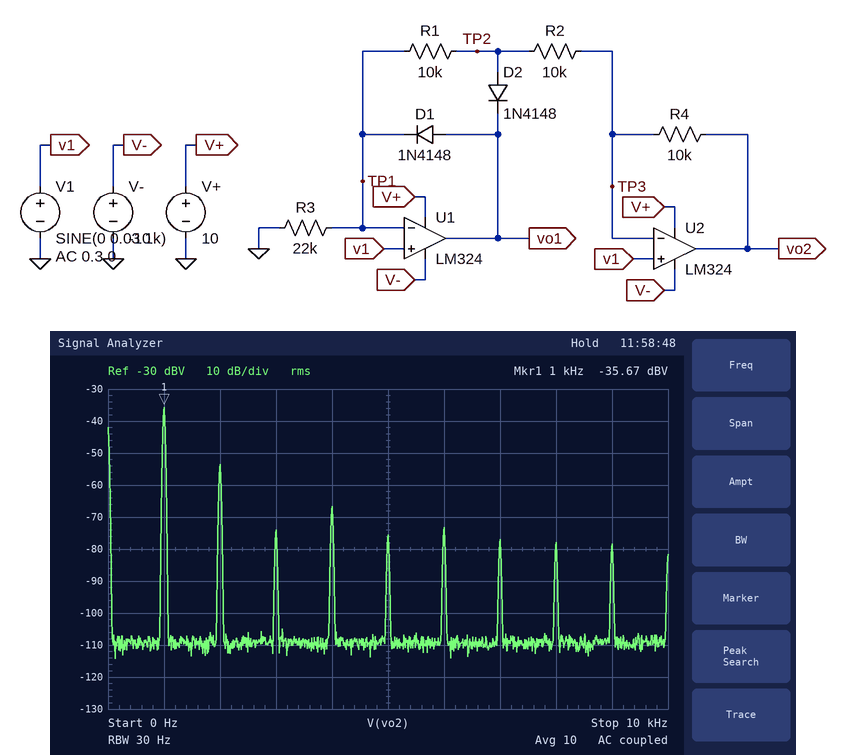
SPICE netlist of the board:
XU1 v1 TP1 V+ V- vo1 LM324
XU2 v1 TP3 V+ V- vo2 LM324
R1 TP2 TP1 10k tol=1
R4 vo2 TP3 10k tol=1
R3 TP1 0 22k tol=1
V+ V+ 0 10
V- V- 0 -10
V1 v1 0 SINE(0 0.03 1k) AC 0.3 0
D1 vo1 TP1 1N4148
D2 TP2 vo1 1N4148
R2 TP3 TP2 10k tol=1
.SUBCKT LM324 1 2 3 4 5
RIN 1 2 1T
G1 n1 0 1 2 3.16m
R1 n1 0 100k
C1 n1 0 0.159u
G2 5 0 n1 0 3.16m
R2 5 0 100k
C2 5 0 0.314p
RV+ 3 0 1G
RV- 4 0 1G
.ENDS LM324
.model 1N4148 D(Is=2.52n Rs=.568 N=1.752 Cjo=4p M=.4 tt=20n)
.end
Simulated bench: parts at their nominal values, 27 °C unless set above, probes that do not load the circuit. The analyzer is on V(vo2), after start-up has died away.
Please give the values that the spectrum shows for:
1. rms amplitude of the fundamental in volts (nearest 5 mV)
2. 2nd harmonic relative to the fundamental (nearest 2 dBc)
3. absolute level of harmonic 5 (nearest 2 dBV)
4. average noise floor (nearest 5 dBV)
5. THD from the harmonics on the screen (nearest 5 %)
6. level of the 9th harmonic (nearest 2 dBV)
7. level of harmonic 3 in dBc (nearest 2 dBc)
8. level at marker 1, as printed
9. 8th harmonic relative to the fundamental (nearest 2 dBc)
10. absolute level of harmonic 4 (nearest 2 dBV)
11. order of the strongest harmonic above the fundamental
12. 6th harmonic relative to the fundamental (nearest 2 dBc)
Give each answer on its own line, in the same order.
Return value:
15 mV
-18 dBc
-76 dBV
-110 dBV
15 %
-78 dBV
-38 dBc
-35.67 dBV
-42 dBc
-66 dBV
2
-38 dBc
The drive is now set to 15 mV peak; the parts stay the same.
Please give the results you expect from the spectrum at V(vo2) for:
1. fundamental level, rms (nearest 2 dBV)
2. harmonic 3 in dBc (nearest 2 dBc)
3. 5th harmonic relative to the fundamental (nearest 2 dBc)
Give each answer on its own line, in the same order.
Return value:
-42 dBV
-34 dBc
-36 dBc
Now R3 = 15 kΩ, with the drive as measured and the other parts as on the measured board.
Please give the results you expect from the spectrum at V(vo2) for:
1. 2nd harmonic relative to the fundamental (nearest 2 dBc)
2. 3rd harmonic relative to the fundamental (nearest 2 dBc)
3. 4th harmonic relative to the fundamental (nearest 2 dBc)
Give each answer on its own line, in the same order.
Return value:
-14 dBc
-36 dBc
-26 dBc
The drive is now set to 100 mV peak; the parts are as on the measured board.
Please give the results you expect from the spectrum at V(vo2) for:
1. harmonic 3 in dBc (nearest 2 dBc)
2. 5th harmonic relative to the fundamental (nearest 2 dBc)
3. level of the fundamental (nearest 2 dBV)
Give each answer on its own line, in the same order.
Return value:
-46 dBc
-48 dBc
-26 dBV
